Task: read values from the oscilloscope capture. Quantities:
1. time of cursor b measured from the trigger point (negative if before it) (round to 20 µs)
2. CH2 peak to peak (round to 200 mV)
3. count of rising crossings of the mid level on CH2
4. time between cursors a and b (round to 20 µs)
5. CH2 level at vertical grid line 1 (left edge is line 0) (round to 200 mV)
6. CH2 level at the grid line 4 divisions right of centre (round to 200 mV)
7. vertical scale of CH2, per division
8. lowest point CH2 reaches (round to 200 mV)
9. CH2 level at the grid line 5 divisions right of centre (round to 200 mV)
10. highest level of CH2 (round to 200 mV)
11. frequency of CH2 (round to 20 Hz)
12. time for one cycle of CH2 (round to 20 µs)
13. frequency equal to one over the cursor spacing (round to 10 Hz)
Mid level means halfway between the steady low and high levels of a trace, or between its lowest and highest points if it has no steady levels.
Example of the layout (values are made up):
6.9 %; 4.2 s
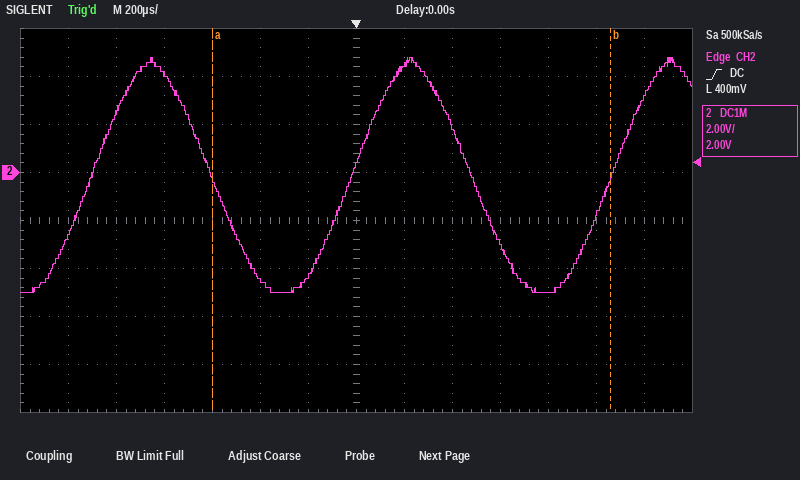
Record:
+1.06 ms; 9.8 V; 3; 1.66 ms; -2.6 V; -5.0 V; 2 V; -5.0 V; -1.8 V; 4.8 V; 920 Hz; 1.08 ms; 600 Hz
